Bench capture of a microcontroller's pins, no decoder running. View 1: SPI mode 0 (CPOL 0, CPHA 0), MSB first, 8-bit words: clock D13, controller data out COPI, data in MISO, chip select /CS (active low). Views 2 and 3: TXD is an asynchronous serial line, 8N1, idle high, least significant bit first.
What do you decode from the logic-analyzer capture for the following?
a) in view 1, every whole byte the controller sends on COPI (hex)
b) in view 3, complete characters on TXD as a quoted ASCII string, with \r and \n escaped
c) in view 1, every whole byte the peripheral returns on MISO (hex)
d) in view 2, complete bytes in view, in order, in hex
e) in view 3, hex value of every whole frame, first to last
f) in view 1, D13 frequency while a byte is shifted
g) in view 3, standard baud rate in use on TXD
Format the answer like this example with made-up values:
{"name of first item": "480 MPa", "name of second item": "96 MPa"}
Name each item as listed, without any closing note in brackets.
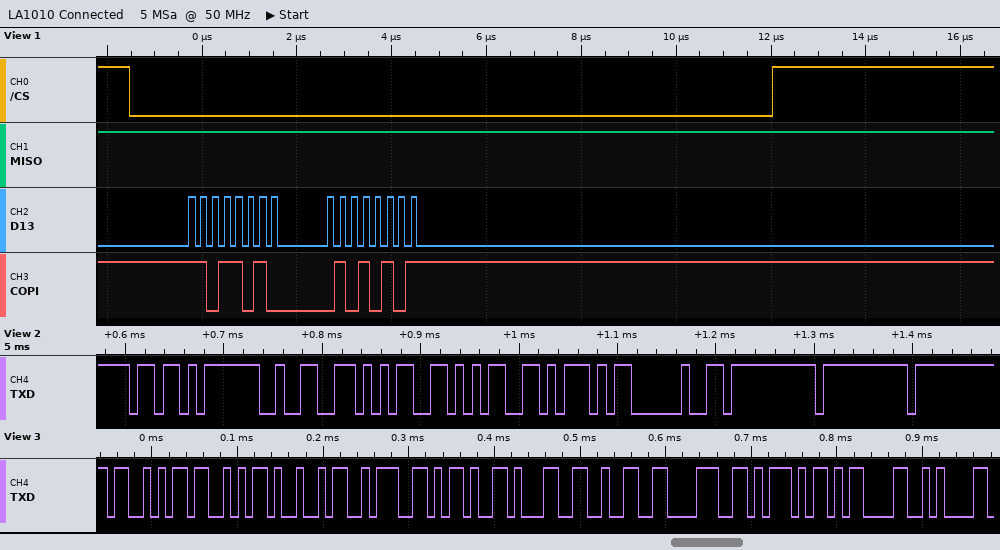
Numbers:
{"in view 1, every whole byte the controller sends on COPI": "DA 55", "in view 3, complete characters on TXD as a quoted ASCII string, with \\r and \\n escaped": "\"SSI:-128]\\r\\n\"", "in view 1, every whole byte the peripheral returns on MISO": "FF FF", "in view 2, complete bytes in view, in order, in hex": "0x5B 0x32 0x35 0x35 0x5D 0x20 0xFF 0xFF 0xFF", "in view 3, hex value of every whole frame, first to last": "53 53 49 3A 2D 31 32 38 5D 0D 0A", "in view 1, D13 frequency while a byte is shifted": "4 MHz", "in view 3, standard baud rate in use on TXD": "115200 baud"}
